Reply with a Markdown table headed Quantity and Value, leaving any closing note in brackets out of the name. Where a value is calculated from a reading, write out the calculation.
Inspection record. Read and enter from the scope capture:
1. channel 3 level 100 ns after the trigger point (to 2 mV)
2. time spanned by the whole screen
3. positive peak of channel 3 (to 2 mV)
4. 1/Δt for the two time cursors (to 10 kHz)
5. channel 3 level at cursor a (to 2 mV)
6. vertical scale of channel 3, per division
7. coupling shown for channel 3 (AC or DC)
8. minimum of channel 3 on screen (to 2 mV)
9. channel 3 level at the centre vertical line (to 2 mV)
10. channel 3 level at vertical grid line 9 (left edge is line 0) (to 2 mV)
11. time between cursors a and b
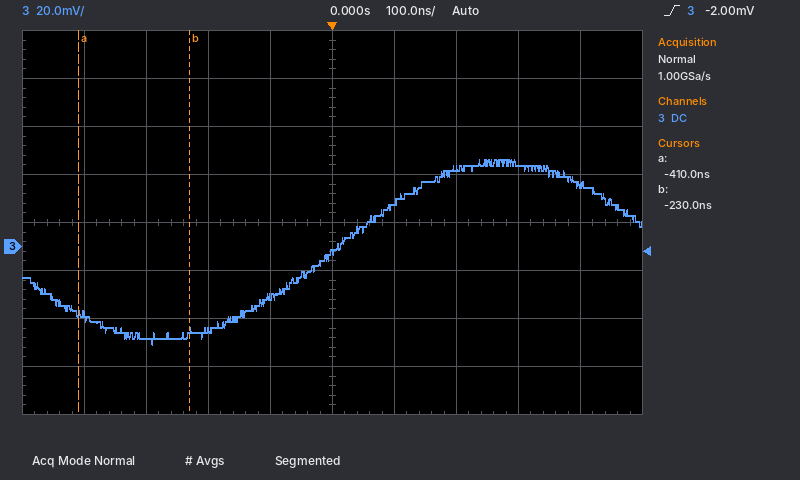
| Quantity | Value |
|---|---|
| channel 3 level 100 ns after the trigger point | 18 mV |
| time spanned by the whole screen | 1 µs |
| positive peak of channel 3 | 36 mV |
| 1/Δt for the two time cursors | 1 / 180 ns ≈ 5.56 MHz |
| channel 3 level at cursor a | -28 mV |
| vertical scale of channel 3, per division | 20 mV |
| coupling shown for channel 3 | DC |
| minimum of channel 3 on screen | -40 mV |
| channel 3 level at the centre vertical line | -2 mV |
| channel 3 level at vertical grid line 9 (left edge is line 0) | 26 mV |
| time between cursors a and b | -230 ns − (-410 ns) = 180 ns |
